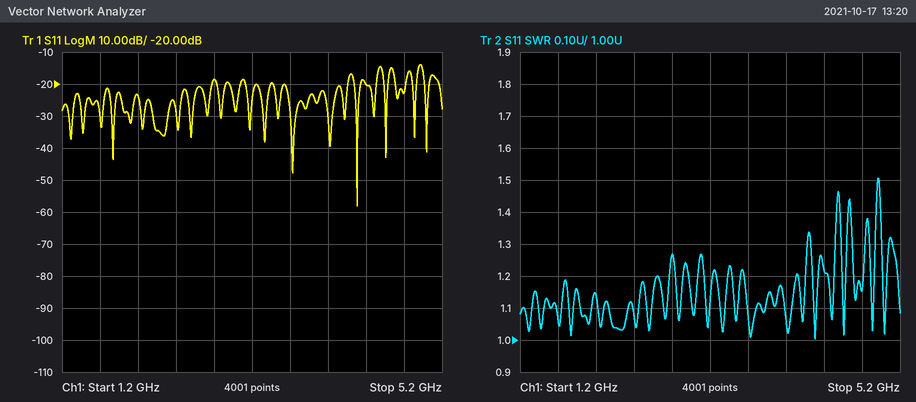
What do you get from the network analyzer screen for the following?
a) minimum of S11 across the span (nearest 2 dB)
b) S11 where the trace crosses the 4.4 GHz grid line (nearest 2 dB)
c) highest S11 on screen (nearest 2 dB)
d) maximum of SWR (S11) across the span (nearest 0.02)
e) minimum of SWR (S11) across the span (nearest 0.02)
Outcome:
-58 dB
-20 dB
-14 dB
1.50
1.00
